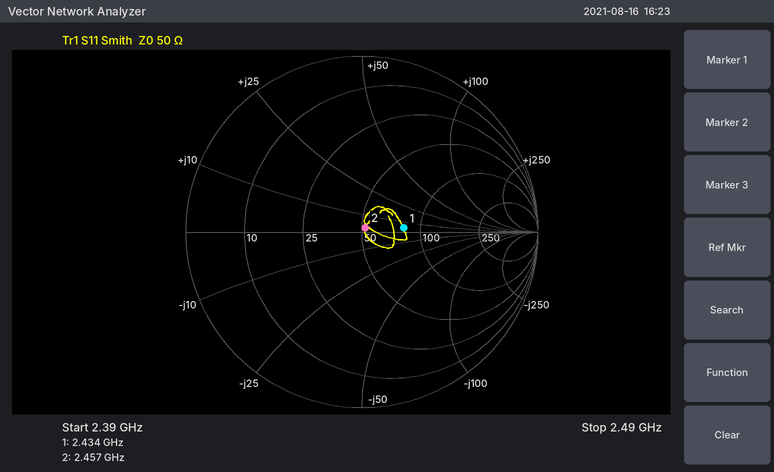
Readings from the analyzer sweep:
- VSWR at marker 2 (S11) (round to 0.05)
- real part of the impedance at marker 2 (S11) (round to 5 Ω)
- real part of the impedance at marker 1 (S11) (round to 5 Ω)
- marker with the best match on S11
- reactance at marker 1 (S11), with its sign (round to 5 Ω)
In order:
1.05
50 Ω
80 Ω
marker 2
+5 Ω
